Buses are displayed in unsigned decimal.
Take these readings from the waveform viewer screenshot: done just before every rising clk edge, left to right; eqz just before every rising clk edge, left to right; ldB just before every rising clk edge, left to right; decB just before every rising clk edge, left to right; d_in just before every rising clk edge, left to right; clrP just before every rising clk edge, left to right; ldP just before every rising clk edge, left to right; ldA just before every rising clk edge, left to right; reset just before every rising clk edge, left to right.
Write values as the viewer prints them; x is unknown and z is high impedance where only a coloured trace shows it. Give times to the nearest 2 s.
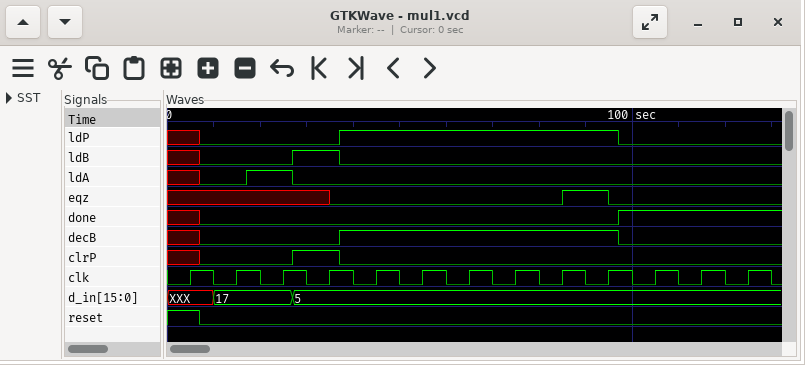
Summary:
x 0 0 0 0 0 0 0 0 0 1 1 1
x x x x 0 0 0 0 0 1 0 0 0
x 0 0 1 0 0 0 0 0 0 0 0 0
x 0 0 0 1 1 1 1 1 1 0 0 0
XXX, 17, 17, 5, 5, 5, 5, 5, 5, 5, 5, 5, 5
x 0 0 1 0 0 0 0 0 0 0 0 0
x 0 0 0 1 1 1 1 1 1 0 0 0
x 0 1 0 0 0 0 0 0 0 0 0 0
1 0 0 0 0 0 0 0 0 0 0 0 0
